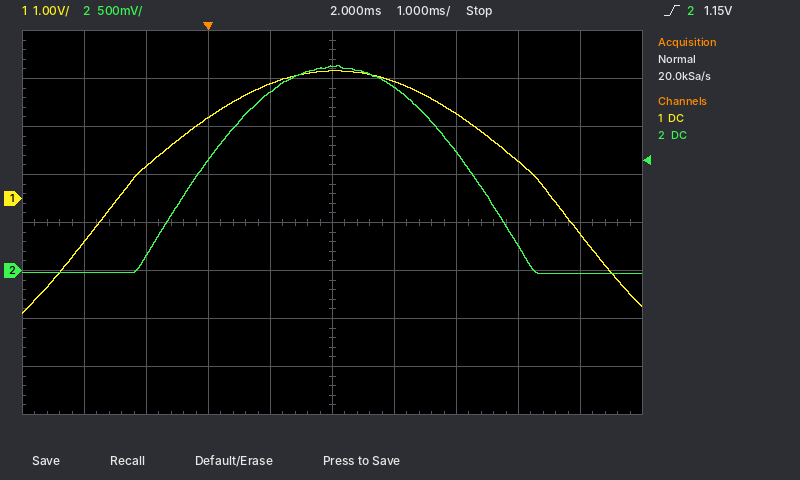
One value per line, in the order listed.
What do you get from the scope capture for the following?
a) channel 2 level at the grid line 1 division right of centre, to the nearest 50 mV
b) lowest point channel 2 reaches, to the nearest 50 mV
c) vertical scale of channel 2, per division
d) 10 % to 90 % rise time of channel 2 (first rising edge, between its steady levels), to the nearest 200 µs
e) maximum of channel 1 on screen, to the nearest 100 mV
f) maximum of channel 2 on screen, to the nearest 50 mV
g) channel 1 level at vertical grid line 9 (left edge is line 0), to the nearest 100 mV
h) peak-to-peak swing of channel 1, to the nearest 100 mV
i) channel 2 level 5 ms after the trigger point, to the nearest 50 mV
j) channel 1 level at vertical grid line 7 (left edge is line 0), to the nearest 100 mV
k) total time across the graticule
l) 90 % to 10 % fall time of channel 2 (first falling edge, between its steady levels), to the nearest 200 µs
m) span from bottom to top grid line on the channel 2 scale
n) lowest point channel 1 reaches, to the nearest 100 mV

1.90 V
-50 mV
500 mV
2.0 ms
2.7 V
2.15 V
-700 mV
5.1 V
250 mV
1.8 V
10 ms
2.0 ms
4 V
-2.4 V
